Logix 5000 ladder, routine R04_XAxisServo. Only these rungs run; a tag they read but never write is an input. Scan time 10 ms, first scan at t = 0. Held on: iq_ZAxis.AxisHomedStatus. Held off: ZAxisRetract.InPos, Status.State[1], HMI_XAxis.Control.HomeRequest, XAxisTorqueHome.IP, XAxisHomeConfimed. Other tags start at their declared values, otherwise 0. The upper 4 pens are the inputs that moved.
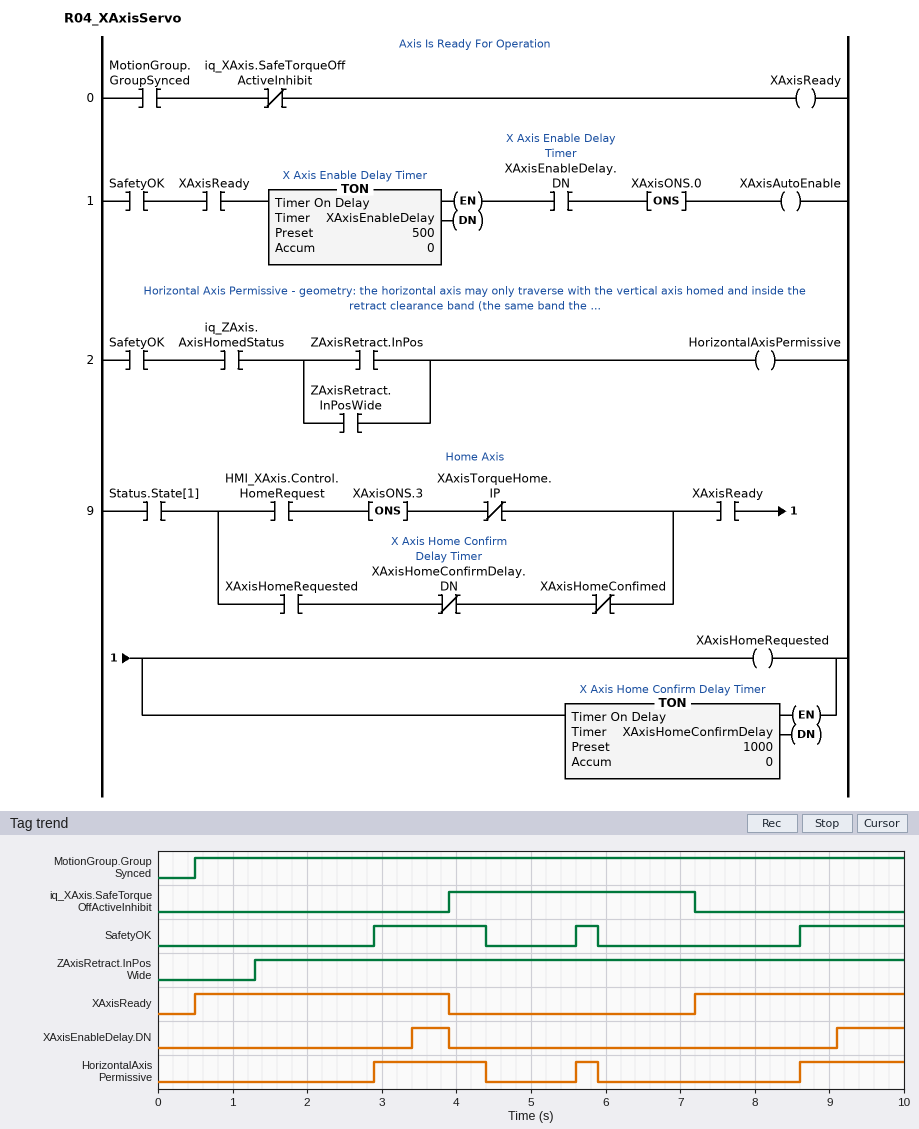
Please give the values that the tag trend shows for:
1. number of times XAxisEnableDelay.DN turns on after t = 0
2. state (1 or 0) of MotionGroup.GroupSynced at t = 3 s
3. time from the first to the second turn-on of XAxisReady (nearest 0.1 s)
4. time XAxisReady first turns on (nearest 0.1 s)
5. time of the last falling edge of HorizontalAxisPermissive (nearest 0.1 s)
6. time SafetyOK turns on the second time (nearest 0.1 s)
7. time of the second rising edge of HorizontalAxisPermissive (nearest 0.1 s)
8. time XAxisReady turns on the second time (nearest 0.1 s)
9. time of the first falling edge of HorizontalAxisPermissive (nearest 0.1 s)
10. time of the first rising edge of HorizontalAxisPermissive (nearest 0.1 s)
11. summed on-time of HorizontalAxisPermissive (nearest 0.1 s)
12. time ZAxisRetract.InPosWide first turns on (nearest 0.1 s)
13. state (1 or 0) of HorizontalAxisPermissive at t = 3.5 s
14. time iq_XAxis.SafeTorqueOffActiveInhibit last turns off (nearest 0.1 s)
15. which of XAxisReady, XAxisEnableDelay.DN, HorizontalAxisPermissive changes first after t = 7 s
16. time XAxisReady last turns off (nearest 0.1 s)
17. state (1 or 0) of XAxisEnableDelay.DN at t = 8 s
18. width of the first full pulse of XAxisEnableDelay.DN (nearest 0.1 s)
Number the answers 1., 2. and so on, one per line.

1. 2
2. 1
3. 6.7 s
4. 0.5 s
5. 5.9 s
6. 5.6 s
7. 5.6 s
8. 7.2 s
9. 4.4 s
10. 2.9 s
11. 3.2 s
12. 1.3 s
13. 1
14. 7.2 s
15. XAxisReady
16. 3.9 s
17. 0
18. 0.5 s
